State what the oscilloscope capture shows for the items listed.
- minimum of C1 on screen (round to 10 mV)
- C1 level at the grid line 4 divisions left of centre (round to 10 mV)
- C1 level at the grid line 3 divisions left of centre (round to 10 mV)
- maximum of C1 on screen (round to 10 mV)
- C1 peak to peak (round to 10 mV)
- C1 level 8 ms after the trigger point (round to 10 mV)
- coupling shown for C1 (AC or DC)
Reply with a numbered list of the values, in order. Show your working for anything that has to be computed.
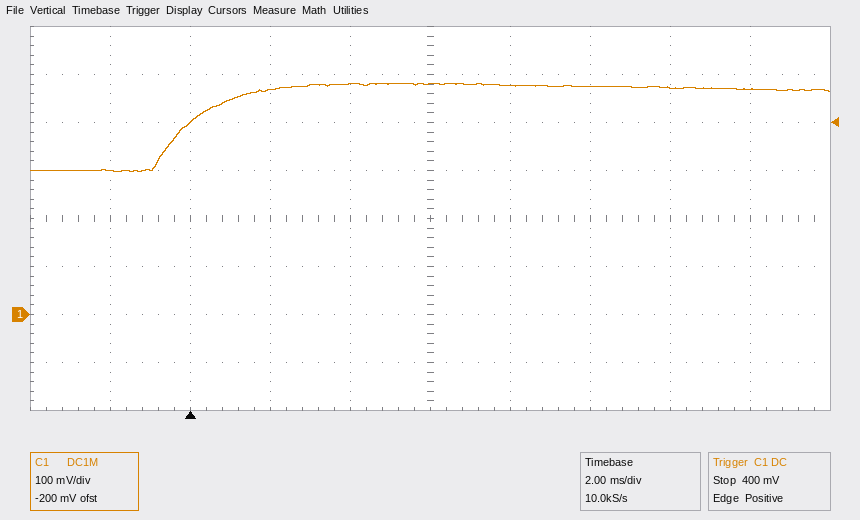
1. 300 mV
2. 300 mV
3. 400 mV
4. 480 mV
5. 480 mV − (300 mV) = 180 mV
6. 480 mV
7. DC
